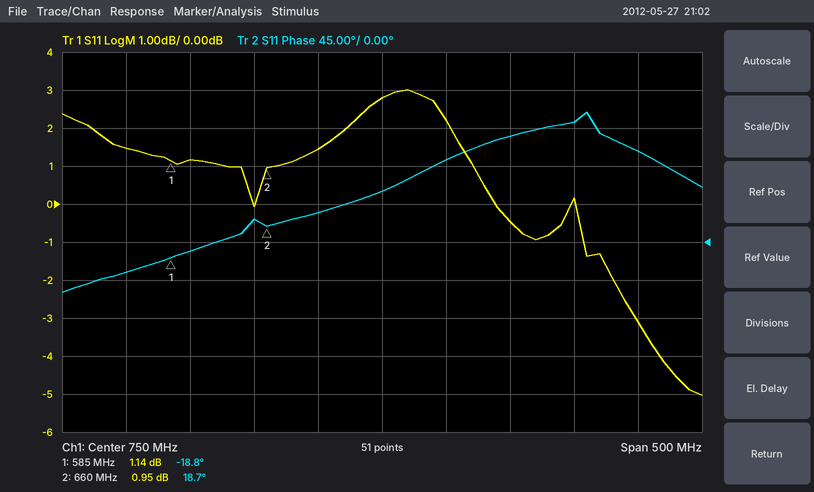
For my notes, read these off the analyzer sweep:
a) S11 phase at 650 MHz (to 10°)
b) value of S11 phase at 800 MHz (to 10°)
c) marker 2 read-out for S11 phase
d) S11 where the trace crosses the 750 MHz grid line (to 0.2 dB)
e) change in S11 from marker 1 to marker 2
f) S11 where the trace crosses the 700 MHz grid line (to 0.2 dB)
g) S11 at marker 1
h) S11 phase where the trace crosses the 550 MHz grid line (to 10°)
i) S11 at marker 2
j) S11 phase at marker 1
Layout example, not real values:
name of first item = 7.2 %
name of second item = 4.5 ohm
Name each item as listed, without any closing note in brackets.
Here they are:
S11 phase at 650 MHz = 30°
value of S11 phase at 800 MHz = 100°
marker 2 read-out for S11 phase = 18.7°
S11 where the trace crosses the 750 MHz grid line = 2.8 dB
change in S11 from marker 1 to marker 2 = -0.19 dB
S11 where the trace crosses the 700 MHz grid line = 1.4 dB
S11 at marker 1 = 1.14 dB
S11 phase where the trace crosses the 550 MHz grid line = -40°
S11 at marker 2 = 0.95 dB
S11 phase at marker 1 = -18.8°
